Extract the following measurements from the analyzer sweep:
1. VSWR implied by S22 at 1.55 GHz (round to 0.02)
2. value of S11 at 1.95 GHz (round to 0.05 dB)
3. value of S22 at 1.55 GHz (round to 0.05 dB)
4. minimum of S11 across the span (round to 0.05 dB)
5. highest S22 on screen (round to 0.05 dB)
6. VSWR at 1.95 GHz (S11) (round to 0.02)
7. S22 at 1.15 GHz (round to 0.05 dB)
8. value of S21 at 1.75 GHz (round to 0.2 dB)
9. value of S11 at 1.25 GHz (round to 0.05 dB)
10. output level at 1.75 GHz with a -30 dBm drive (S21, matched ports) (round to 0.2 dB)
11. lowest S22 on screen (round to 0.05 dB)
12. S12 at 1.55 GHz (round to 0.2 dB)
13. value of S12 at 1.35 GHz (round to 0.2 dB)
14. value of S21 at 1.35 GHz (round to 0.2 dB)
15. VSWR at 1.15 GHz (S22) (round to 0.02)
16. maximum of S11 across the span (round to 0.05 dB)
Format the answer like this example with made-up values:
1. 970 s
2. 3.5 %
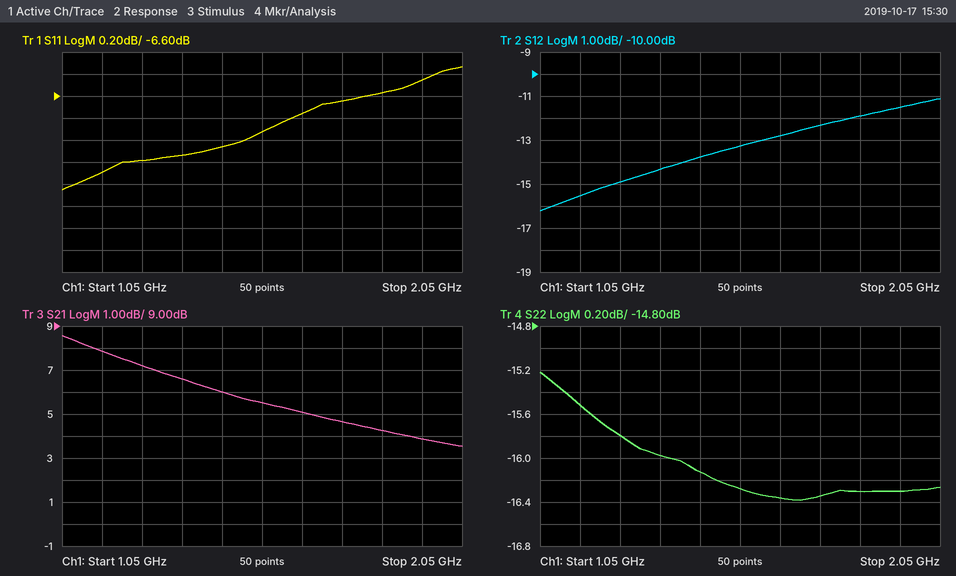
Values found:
1. 1.36
2. -6.45 dB
3. -16.30 dB
4. -7.45 dB
5. -15.20 dB
6. 2.82
7. -15.50 dB
8. 4.6 dB
9. -7.20 dB
10. -25.4 dBm
11. -16.40 dB
12. -13.2 dB
13. -14.4 dB
14. 6.6 dB
15. 1.40
16. -6.35 dB
